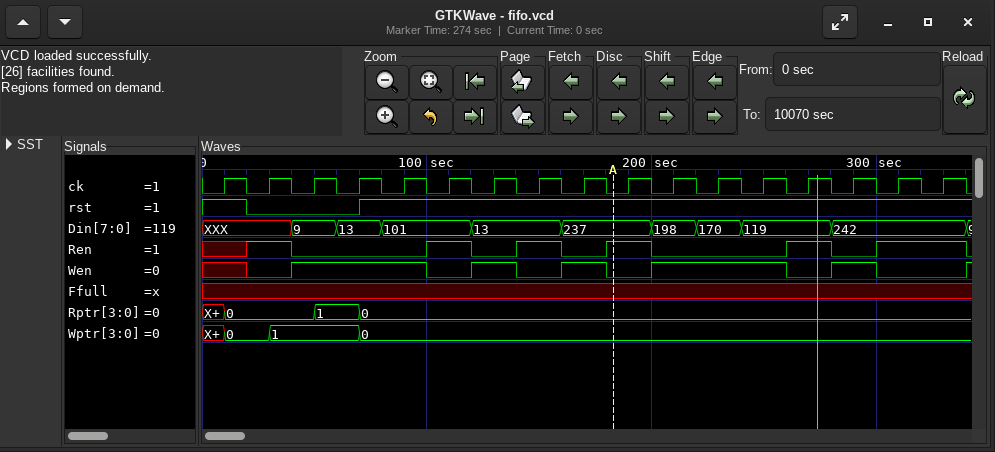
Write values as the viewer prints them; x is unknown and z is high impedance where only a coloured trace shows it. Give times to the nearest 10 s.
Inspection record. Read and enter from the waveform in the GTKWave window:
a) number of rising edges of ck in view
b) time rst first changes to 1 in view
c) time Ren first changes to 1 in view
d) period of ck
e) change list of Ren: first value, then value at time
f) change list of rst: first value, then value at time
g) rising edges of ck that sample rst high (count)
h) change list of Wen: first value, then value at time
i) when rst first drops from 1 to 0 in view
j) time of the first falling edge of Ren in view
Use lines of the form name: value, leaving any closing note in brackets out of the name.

number of rising edges of ck in view: 17
time rst first changes to 1 in view: 70 s
time Ren first changes to 1 in view: 20 s
period of ck: 20 s
change list of Ren: first value, then value at time: x, 1 at 20 s, 0 at 40 s, 1 at 100 s, 0 at 120 s, 1 at 140 s, 0 at 160 s, 1 at 180 s, 0 at 200 s, 1 at 260 s, 0 at 280 s, 1 at 300 s, 0 at 340 s
change list of rst: first value, then value at time: 1, 0 at 20 s, 1 at 70 s
rising edges of ck that sample rst high: 14
change list of Wen: first value, then value at time: x, 0 at 20 s, 1 at 40 s, 0 at 100 s, 1 at 120 s, 0 at 140 s, 1 at 160 s, 0 at 180 s, 1 at 200 s, 0 at 260 s, 1 at 280 s, 0 at 300 s, 1 at 340 s
when rst first drops from 1 to 0 in view: 20 s
time of the first falling edge of Ren in view: 40 s
